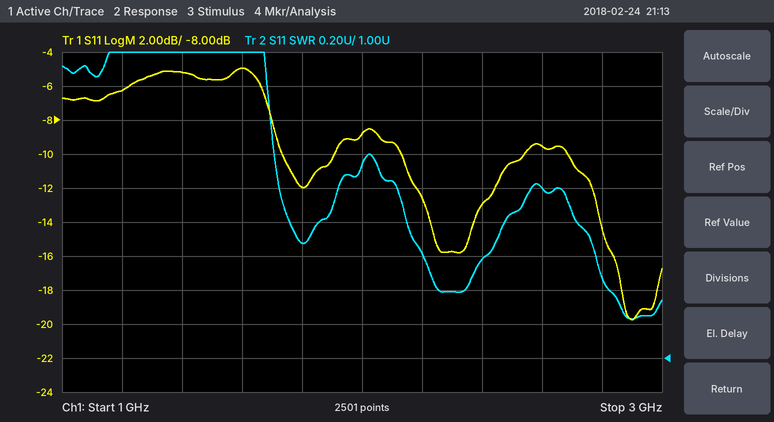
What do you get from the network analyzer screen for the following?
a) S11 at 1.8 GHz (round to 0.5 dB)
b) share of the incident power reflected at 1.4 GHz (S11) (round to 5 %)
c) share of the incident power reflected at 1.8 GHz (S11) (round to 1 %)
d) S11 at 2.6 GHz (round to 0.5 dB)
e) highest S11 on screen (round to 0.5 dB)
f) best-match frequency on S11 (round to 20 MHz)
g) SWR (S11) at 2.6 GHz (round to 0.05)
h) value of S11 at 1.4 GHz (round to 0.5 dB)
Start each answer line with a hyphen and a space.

- -12.0 dB
- 30 %
- 6 %
- -9.5 dB
- -5.0 dB
- 2.90 GHz
- 2.00
- -5.0 dB
